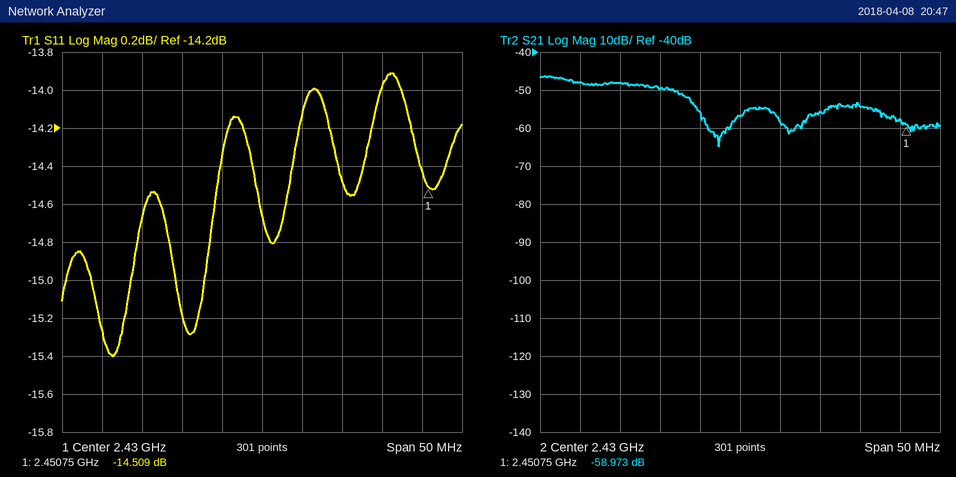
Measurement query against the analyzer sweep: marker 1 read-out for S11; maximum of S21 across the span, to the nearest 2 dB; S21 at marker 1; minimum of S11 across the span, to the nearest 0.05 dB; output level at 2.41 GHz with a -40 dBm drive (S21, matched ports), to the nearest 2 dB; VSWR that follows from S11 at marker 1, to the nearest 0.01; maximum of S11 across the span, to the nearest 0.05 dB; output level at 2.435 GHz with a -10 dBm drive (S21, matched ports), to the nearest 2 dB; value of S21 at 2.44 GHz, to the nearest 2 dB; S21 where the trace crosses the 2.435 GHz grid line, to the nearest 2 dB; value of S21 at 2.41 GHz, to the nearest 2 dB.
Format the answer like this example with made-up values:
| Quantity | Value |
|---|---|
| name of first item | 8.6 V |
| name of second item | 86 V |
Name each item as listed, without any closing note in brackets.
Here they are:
| Quantity | Value |
|---|---|
| marker 1 read-out for S11 | -14.509 dB |
| maximum of S21 across the span, to the nearest 2 dB | -46 dB |
| S21 at marker 1 | -58.973 dB |
| minimum of S11 across the span, to the nearest 0.05 dB | -15.40 dB |
| output level at 2.41 GHz with a -40 dBm drive (S21, matched ports), to the nearest 2 dB | -88 dBm |
| VSWR that follows from S11 at marker 1, to the nearest 0.01 | 1.46 |
| maximum of S11 across the span, to the nearest 0.05 dB | -13.90 dB |
| output level at 2.435 GHz with a -10 dBm drive (S21, matched ports), to the nearest 2 dB | -68 dBm |
| value of S21 at 2.44 GHz, to the nearest 2 dB | -56 dB |
| S21 where the trace crosses the 2.435 GHz grid line, to the nearest 2 dB | -58 dB |
| value of S21 at 2.41 GHz, to the nearest 2 dB | -48 dB |
